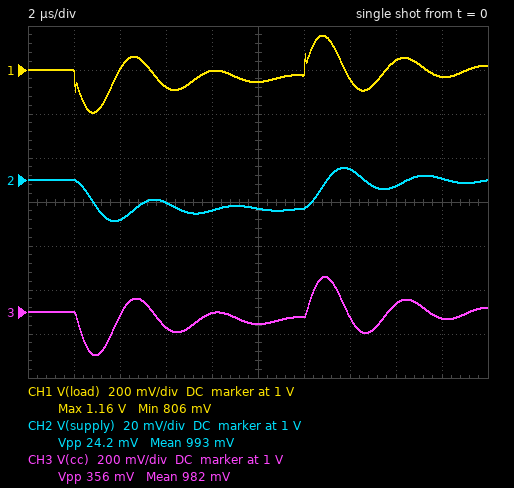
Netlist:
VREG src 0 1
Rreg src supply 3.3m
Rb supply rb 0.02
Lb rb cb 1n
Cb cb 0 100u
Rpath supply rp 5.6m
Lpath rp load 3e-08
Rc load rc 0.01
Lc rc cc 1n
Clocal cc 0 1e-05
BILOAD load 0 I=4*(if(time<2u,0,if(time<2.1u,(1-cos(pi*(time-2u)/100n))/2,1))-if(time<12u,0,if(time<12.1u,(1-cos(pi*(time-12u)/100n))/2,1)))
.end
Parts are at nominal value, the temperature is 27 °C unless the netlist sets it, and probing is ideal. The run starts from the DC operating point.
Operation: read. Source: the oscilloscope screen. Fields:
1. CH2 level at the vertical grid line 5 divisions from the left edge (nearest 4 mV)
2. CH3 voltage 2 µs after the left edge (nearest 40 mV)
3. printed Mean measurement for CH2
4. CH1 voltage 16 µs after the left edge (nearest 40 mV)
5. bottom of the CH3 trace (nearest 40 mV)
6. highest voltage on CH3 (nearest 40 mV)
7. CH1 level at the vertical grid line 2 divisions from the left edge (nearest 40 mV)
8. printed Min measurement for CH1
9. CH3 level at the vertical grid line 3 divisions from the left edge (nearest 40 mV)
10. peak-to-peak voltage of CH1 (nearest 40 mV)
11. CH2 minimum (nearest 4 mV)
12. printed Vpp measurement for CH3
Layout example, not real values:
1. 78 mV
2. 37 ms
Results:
1. 988 mV
2. 1.00 V
3. 993 mV
4. 1.04 V
5. 800 mV
6. 1.16 V
7. 1.00 V
8. 806 mV
9. 920 mV
10. 360 mV
11. 980 mV
12. 356 mV
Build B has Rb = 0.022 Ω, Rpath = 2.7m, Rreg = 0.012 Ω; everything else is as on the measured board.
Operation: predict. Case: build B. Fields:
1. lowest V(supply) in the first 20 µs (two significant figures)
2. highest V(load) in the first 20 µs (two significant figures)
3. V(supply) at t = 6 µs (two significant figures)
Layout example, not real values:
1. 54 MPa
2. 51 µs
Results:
1. 950 mV
2. 1.1 V
3. 960 mV
